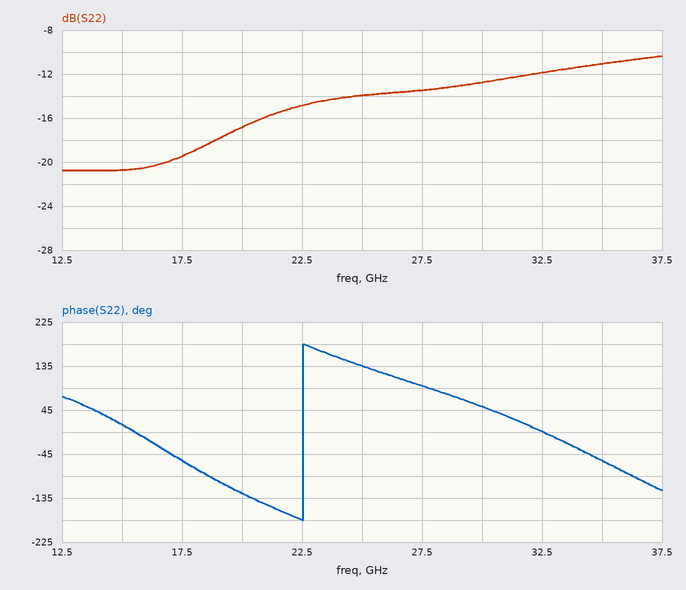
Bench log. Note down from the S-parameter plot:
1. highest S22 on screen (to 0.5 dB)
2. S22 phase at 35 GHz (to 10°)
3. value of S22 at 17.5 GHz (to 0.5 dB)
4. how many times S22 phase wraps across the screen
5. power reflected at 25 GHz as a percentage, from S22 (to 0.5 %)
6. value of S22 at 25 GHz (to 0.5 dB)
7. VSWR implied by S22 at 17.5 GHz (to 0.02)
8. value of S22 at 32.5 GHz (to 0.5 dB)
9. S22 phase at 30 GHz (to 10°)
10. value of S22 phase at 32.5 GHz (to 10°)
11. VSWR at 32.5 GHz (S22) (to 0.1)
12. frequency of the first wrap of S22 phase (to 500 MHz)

-10.5 dB
-60°
-19.5 dB
1
4.0 %
-14.0 dB
1.24
-12.0 dB
50°
0°
1.7
22.5 GHz
